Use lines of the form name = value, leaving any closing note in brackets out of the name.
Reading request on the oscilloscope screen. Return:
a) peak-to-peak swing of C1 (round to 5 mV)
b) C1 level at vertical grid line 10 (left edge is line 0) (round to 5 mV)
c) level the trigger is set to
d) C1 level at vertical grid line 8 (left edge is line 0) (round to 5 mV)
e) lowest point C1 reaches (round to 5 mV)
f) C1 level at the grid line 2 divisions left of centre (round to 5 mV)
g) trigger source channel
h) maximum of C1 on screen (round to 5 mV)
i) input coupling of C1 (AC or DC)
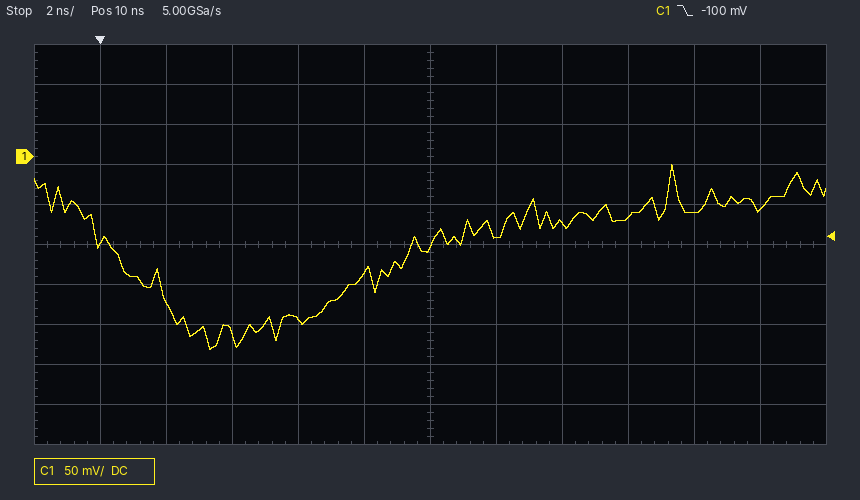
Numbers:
peak-to-peak swing of C1 = 230 mV
C1 level at vertical grid line 10 (left edge is line 0) = -70 mV
level the trigger is set to = -100 mV
C1 level at vertical grid line 8 (left edge is line 0) = -85 mV
lowest point C1 reaches = -240 mV
C1 level at the grid line 2 divisions left of centre = -205 mV
trigger source channel = C1
maximum of C1 on screen = -10 mV
input coupling of C1 = DC
